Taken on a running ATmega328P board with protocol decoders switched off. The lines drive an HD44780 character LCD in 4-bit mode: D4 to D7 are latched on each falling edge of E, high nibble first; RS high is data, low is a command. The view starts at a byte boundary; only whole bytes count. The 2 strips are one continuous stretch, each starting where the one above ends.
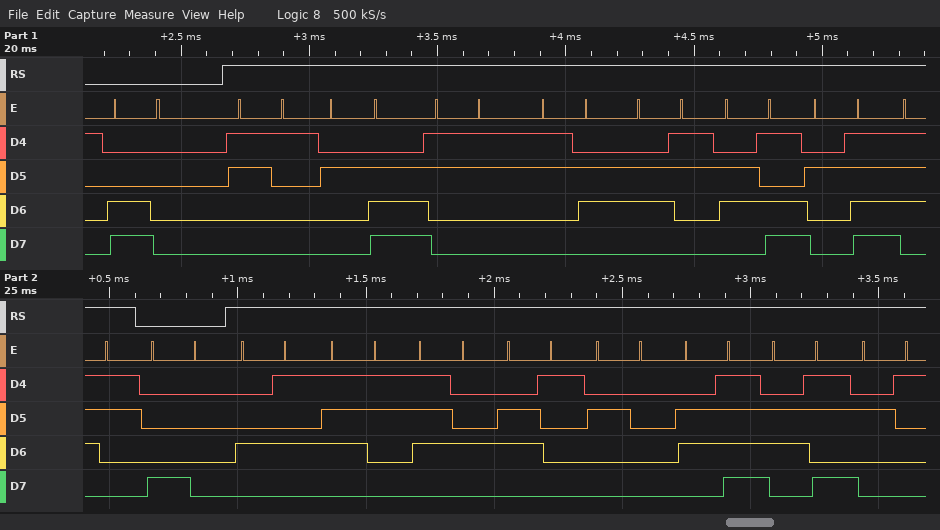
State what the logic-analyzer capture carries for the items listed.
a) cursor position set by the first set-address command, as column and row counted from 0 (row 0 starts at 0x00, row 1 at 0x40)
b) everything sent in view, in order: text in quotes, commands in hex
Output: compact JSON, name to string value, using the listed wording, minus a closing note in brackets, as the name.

{"cursor position set by the first set-address command, as column and row counted from 0": "column 0, row 1", "everything sent in view, in order: text in quotes, commands in hex": "0xC0 \"1.36cm/s\" 0x80 \"Esta ok!\""}
